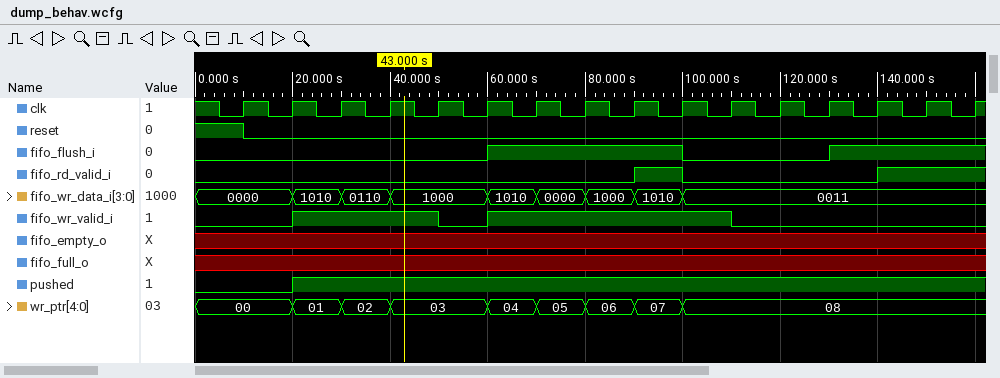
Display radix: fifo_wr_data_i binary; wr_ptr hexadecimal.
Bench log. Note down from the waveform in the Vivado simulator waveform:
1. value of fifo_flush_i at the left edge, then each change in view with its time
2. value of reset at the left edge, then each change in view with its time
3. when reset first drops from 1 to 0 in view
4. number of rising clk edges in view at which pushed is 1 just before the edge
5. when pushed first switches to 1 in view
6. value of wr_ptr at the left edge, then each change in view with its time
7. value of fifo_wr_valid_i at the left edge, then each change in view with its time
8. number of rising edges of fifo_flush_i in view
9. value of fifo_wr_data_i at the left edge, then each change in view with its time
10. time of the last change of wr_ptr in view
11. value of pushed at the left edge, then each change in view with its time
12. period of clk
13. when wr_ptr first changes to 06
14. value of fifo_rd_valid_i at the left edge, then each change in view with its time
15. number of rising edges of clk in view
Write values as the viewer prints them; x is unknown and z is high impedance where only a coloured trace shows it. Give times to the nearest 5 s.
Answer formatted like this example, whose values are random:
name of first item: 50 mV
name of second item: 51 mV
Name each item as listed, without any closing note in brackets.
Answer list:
value of fifo_flush_i at the left edge, then each change in view with its time: 0, 1 at 60 s, 0 at 100 s, 1 at 130 s
value of reset at the left edge, then each change in view with its time: 1, 0 at 10 s
when reset first drops from 1 to 0 in view: 10 s
number of rising clk edges in view at which pushed is 1 just before the edge: 14
when pushed first switches to 1 in view: 20 s
value of wr_ptr at the left edge, then each change in view with its time: 00, 01 at 20 s, 02 at 30 s, 03 at 40 s, 04 at 60 s, 05 at 70 s, 06 at 80 s, 07 at 90 s, 08 at 100 s
value of fifo_wr_valid_i at the left edge, then each change in view with its time: 0, 1 at 20 s, 0 at 50 s, 1 at 60 s, 0 at 110 s
number of rising edges of fifo_flush_i in view: 2
value of fifo_wr_data_i at the left edge, then each change in view with its time: 0000, 1010 at 20 s, 0110 at 30 s, 1000 at 40 s, 1010 at 60 s, 0000 at 70 s, 1000 at 80 s, 1010 at 90 s, 0011 at 100 s
time of the last change of wr_ptr in view: 100 s
value of pushed at the left edge, then each change in view with its time: 0, 1 at 20 s
period of clk: 10 s
when wr_ptr first changes to 06: 80 s
value of fifo_rd_valid_i at the left edge, then each change in view with its time: 0, 1 at 90 s, 0 at 100 s, 1 at 140 s
number of rising edges of clk in view: 16
